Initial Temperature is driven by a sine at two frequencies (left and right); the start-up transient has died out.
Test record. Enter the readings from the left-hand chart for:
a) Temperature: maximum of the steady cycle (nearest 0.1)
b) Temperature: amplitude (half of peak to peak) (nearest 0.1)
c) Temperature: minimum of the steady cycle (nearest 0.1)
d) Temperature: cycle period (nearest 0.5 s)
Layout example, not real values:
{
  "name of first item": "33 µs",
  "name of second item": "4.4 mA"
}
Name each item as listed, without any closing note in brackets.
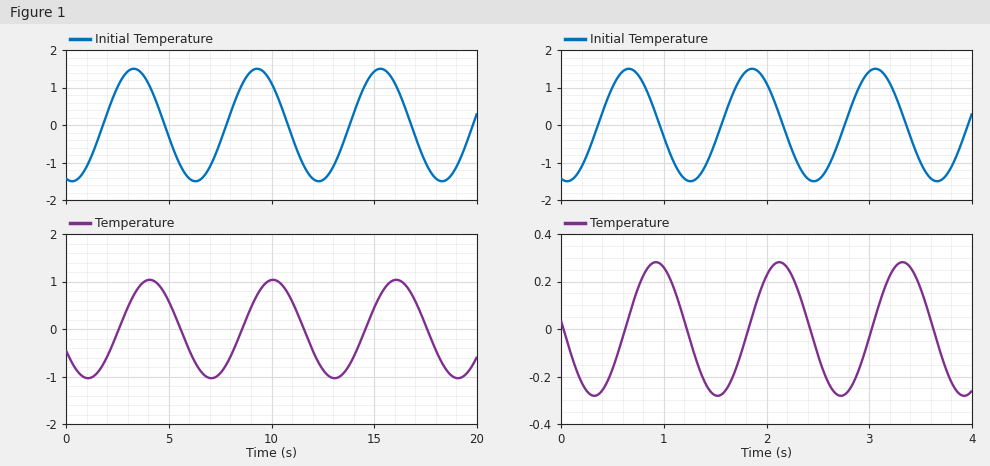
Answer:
{
  "Temperature: maximum of the steady cycle": "1.0",
  "Temperature: amplitude (half of peak to peak)": "1.0",
  "Temperature: minimum of the steady cycle": "-1.0",
  "Temperature: cycle period": "6.0 s"
}
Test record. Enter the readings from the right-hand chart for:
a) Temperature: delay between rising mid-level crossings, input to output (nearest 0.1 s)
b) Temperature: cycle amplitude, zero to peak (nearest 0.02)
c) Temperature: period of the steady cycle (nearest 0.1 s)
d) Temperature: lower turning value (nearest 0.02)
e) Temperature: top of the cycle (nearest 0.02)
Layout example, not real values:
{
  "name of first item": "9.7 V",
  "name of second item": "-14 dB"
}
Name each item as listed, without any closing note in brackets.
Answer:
{
  "Temperature: delay between rising mid-level crossings, input to output": "0.3 s",
  "Temperature: cycle amplitude, zero to peak": "0.28",
  "Temperature: period of the steady cycle": "1.2 s",
  "Temperature: lower turning value": "-0.28",
  "Temperature: top of the cycle": "0.28"
}
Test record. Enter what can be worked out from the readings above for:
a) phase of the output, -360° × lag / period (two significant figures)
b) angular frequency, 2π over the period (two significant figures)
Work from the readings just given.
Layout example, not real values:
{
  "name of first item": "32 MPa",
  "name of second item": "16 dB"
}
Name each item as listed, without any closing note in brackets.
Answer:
{
  "phase of the output, -360° × lag / period": "-90°",
  "angular frequency, 2π over the period": "5.2 rad/s"
}
